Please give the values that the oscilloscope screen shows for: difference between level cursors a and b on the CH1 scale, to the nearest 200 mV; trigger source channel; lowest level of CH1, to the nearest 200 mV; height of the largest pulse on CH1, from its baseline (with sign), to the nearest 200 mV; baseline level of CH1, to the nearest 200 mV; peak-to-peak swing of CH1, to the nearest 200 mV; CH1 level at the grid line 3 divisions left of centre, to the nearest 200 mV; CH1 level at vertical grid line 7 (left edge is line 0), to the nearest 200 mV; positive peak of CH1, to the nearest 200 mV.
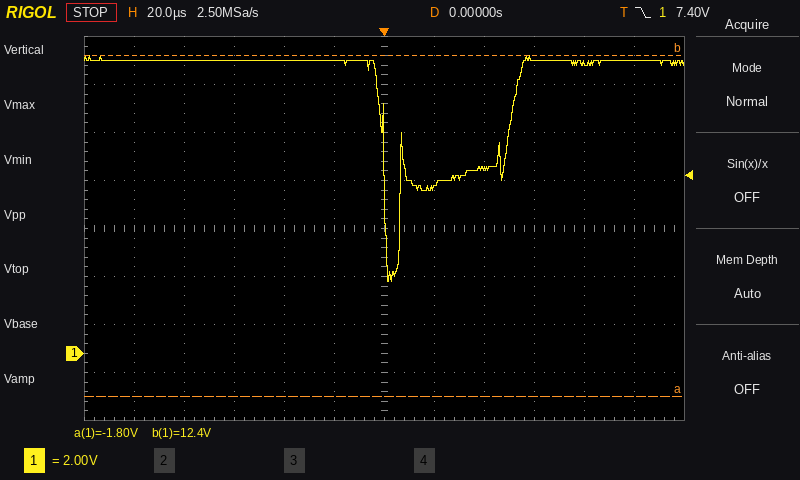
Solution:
14.2 V
CH1
3.0 V
-9.2 V
12.2 V
9.4 V
12.2 V
7.0 V
12.4 V
